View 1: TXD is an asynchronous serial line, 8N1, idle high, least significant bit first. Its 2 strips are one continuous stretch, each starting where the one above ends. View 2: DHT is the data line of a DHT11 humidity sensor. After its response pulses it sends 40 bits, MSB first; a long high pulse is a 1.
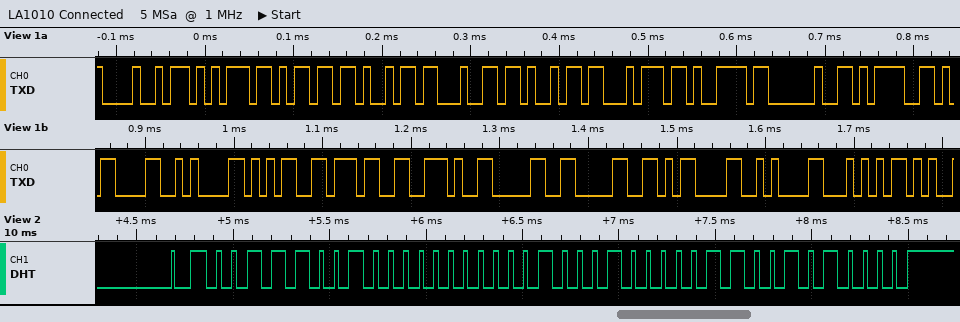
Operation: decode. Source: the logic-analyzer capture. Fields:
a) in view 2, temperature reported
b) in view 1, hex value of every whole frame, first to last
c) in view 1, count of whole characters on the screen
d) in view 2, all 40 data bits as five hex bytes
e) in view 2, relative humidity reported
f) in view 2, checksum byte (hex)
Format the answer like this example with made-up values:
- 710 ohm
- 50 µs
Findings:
- 17.6 °C
- 48 75 6D 69 64 69 74 79 20 3D 0D 0A 35 37 2E 30 30 0D 0A 54
- 20
- 39 00 11 06 50
- 57 %
- 0x50
